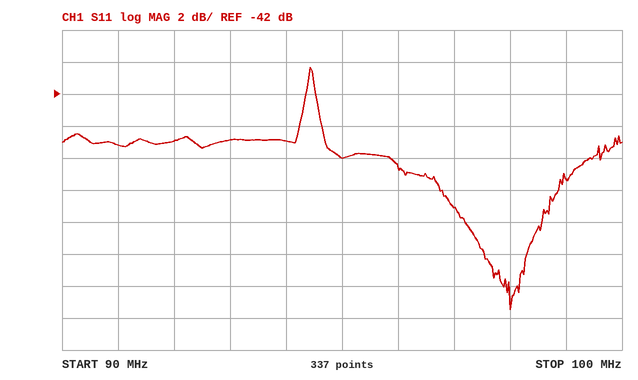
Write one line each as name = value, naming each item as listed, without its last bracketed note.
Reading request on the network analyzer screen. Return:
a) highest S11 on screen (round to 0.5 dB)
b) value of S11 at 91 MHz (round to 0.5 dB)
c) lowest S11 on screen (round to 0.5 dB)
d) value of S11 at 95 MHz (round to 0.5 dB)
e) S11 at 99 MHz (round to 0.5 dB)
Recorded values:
highest S11 on screen = -40.5 dB
value of S11 at 91 MHz = -45.0 dB
lowest S11 on screen = -55.5 dB
value of S11 at 95 MHz = -46.0 dB
S11 at 99 MHz = -47.5 dB
